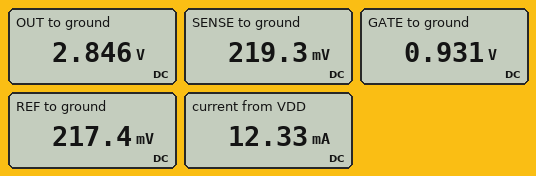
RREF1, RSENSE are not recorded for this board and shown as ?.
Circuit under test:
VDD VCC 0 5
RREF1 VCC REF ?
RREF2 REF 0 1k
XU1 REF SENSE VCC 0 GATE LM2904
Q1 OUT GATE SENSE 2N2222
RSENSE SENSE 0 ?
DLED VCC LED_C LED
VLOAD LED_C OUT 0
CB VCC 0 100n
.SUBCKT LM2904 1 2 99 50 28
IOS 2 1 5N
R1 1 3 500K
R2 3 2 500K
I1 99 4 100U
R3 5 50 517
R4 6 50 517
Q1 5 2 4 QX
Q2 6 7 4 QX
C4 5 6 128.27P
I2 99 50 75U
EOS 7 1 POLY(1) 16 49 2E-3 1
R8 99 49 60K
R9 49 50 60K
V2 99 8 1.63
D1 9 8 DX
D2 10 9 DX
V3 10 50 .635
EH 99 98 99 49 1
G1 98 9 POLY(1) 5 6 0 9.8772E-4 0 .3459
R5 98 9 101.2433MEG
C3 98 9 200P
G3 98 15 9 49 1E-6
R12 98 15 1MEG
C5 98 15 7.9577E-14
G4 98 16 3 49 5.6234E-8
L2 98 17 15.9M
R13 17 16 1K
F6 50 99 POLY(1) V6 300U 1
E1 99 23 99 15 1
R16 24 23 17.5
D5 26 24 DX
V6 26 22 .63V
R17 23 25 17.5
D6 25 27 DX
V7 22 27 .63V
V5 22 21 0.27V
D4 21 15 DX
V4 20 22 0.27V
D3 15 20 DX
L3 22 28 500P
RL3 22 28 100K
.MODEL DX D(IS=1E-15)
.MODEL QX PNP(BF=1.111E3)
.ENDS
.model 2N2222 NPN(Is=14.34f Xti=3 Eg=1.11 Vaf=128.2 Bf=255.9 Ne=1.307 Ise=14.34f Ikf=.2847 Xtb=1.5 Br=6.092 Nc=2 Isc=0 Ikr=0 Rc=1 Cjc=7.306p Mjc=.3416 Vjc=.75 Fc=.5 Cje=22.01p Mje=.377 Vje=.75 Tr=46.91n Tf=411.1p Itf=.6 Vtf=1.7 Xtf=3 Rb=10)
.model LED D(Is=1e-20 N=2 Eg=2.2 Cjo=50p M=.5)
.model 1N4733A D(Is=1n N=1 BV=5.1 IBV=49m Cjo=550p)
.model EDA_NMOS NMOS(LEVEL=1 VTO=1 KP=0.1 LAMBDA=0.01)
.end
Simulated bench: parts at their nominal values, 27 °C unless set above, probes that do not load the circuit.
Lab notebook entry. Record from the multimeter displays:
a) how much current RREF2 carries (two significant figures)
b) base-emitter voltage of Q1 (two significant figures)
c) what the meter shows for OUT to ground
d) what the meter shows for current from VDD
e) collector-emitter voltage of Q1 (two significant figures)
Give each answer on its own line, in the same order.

220 µA
710 mV
2.846 V
12.33 mA
2.6 V
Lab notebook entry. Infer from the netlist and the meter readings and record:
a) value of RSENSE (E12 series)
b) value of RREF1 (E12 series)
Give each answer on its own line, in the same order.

18 Ω
22 kΩ
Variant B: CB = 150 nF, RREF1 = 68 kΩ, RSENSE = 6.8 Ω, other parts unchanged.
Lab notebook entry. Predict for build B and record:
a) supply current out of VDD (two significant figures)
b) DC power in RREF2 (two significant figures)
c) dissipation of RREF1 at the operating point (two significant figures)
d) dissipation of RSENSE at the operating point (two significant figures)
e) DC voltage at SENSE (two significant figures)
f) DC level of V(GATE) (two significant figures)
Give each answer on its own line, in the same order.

11 mA
5.3 µW
360 µW
810 µW
74 mV
780 mV
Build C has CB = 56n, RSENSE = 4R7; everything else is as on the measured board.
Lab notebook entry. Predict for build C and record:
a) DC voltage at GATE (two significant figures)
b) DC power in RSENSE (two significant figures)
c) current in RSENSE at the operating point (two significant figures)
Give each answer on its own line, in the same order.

970 mV
10 mW
47 mA
